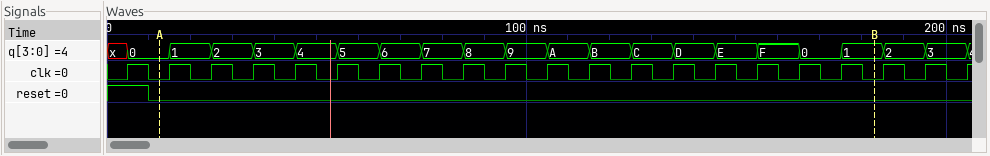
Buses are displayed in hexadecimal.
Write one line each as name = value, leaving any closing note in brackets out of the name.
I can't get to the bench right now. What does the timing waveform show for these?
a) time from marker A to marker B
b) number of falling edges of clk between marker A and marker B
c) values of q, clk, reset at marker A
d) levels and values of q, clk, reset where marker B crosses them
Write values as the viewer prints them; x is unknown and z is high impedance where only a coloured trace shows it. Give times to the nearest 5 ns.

time from marker A to marker B = 170 ns
number of falling edges of clk between marker A and marker B = 17
values of q, clk, reset at marker A = q=0, clk=0, reset=0
levels and values of q, clk, reset where marker B crosses them = q=1, clk=0, reset=0
